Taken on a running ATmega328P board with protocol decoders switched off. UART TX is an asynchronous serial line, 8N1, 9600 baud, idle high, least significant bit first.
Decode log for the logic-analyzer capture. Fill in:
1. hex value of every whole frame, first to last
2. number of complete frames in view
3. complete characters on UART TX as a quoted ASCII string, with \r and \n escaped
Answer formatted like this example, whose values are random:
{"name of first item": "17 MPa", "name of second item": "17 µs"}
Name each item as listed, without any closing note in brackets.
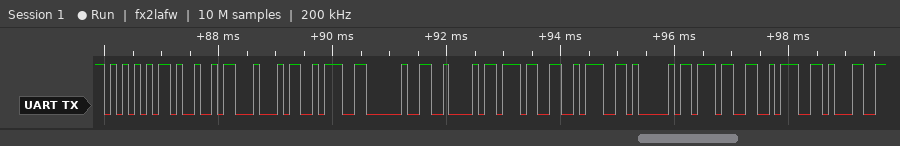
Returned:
{"hex value of every whole frame, first to last": "55 49 44 3A 20 42 37 3A 41 37 3A 31", "number of complete frames in view": "12", "complete characters on UART TX as a quoted ASCII string, with \\r and \\n escaped": "\"UID: B7:A7:1\""}
